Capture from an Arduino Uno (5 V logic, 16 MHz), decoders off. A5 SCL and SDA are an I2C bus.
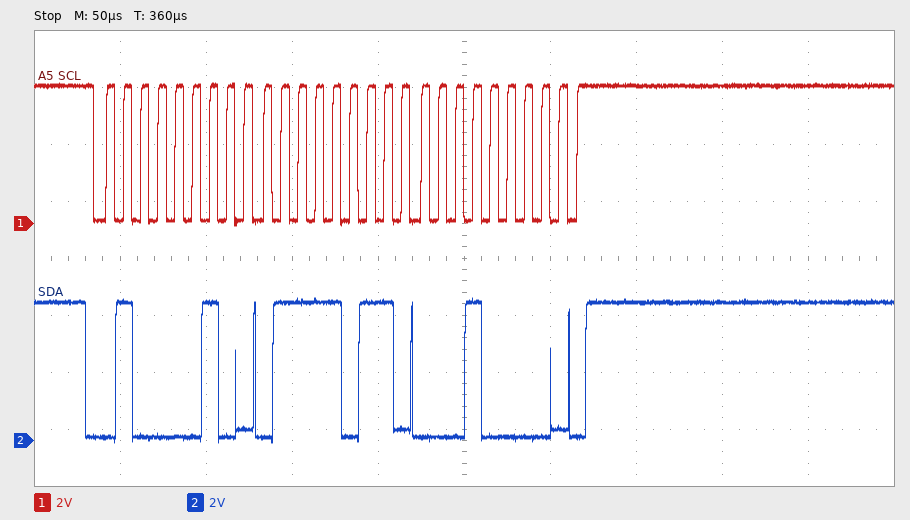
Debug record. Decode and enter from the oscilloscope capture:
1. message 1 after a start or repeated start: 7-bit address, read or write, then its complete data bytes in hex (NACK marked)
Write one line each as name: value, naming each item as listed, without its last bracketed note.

message 1 after a start or repeated start: 7-bit address, read or write, then its complete data bytes in hex: 0x21 write: 7B 10
